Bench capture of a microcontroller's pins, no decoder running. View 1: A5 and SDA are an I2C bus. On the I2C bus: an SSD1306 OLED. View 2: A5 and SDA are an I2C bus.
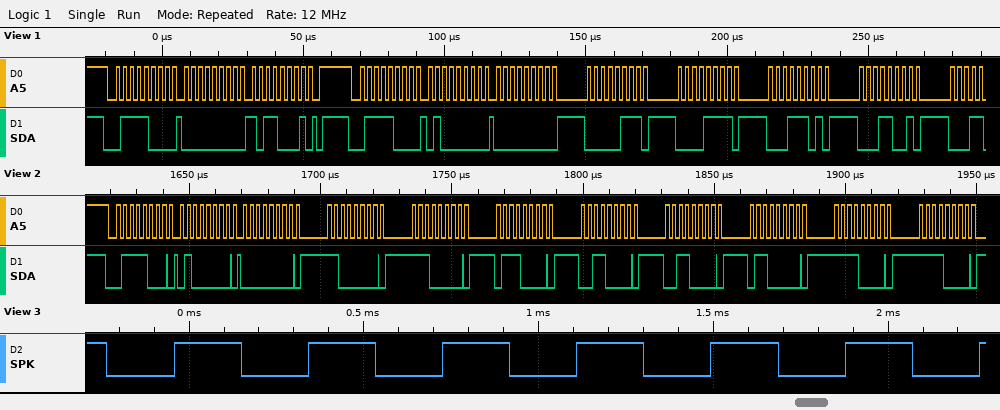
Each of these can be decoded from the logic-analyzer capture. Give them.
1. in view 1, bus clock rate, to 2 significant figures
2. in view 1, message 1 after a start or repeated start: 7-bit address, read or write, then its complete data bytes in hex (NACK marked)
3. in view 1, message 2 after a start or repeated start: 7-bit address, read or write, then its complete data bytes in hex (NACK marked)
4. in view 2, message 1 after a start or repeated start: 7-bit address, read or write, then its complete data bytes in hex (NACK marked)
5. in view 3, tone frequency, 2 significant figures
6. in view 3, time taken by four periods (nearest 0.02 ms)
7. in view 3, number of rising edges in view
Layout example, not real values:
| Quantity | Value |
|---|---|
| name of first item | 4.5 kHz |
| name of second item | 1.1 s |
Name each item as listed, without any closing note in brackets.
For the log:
| Quantity | Value |
|---|---|
| in view 1, bus clock rate, to 2 significant figures | 400 kHz |
| in view 1, message 1 after a start or repeated start: 7-bit address, read or write, then its complete data bytes in hex | 0x3C write: 00 B1 |
| in view 1, message 2 after a start or repeated start: 7-bit address, read or write, then its complete data bytes in hex | 0x3C write: 40 00 07 0F 1D 19 |
| in view 2, message 1 after a start or repeated start: 7-bit address, read or write, then its complete data bytes in hex | 0x3C write: 40 00 C0 E0 70 30 30 60 F0 F0 |
| in view 3, tone frequency, 2 significant figures | 2.6 kHz |
| in view 3, time taken by four periods | 1.54 ms |
| in view 3, number of rising edges in view | 7 |
